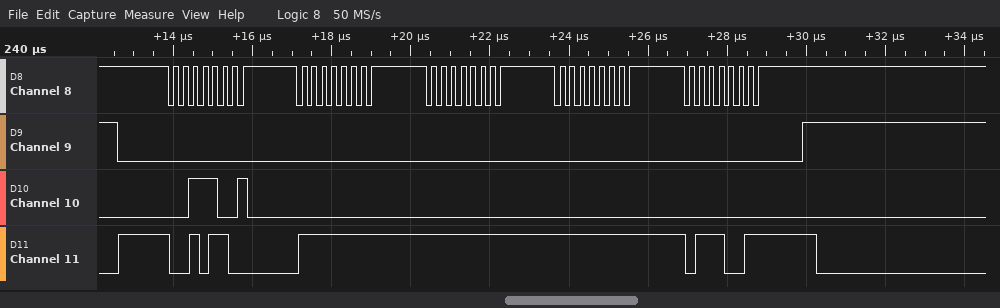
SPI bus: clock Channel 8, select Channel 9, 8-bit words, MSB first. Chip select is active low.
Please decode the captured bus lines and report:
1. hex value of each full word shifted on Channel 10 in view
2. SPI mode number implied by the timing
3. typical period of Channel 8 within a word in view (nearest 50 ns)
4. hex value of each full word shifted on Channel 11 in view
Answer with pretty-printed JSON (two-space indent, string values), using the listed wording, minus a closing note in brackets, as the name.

{
  "hex value of each full word shifted on Channel 10 in view": "39, 00, 00, 00, 00",
  "SPI mode number implied by the timing": "3",
  "typical period of Channel 8 within a word in view": "250 ns",
  "hex value of each full word shifted on Channel 11 in view": "2C, FF, FF, FF, 73"
}
